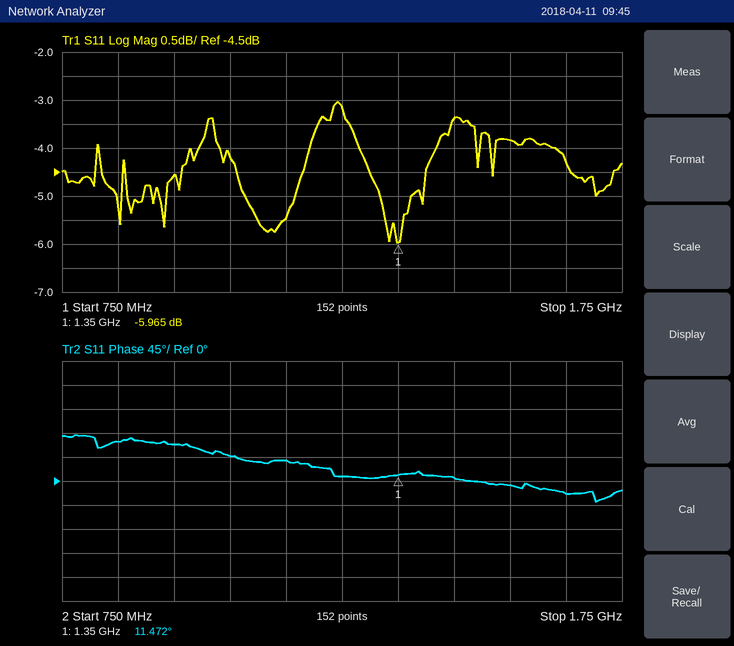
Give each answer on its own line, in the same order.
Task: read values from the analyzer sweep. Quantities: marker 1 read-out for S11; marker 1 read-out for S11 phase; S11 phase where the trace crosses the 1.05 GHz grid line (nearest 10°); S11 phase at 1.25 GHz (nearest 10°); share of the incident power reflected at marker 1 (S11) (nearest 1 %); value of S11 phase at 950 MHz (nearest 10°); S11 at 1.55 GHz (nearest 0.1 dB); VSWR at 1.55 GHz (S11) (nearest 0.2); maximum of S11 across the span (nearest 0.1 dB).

-5.965 dB
11.472°
50°
10°
25 %
70°
-3.8 dB
4.6
-3.0 dB
